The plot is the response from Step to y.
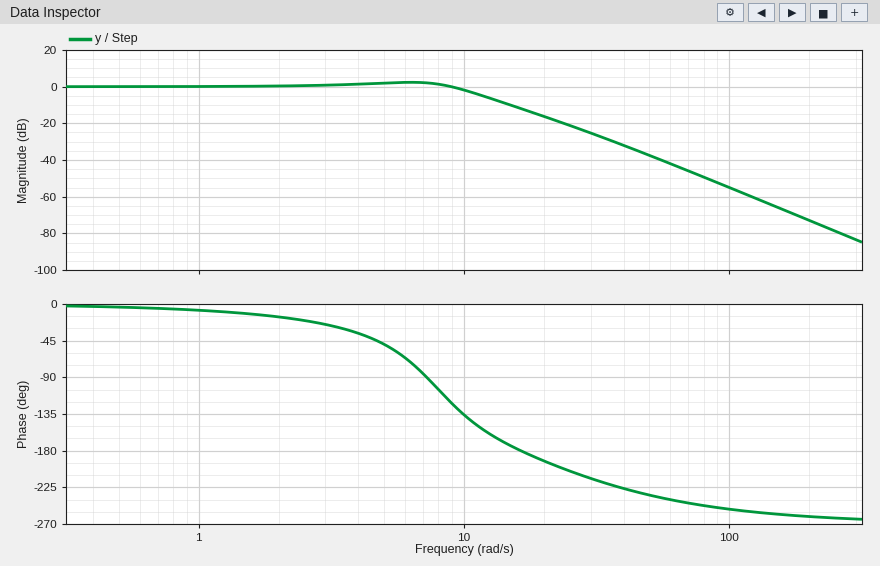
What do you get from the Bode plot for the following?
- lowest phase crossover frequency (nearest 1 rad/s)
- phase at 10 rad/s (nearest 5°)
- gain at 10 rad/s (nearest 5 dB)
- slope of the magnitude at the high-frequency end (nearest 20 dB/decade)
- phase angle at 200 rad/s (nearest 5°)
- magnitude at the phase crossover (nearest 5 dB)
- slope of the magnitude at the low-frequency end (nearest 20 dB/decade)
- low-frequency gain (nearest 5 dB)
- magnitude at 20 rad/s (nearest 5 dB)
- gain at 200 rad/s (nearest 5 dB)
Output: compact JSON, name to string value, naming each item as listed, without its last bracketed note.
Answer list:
{"lowest phase crossover frequency": "16 rad/s", "phase at 10 rad/s": "-135°", "gain at 10 rad/s": "0 dB", "slope of the magnitude at the high-frequency end": "-60 dB/decade", "phase angle at 200 rad/s": "-260°", "magnitude at the phase crossover": "-10 dB", "slope of the magnitude at the low-frequency end": "0 dB/decade", "low-frequency gain": "0 dB", "magnitude at 20 rad/s": "-15 dB", "gain at 200 rad/s": "-75 dB"}
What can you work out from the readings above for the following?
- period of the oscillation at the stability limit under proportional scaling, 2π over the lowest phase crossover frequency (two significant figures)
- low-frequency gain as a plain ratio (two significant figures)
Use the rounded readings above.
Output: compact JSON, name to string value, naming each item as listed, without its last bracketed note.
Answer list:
{"period of the oscillation at the stability limit under proportional scaling, 2π over the lowest phase crossover frequency": "0.39 s", "low-frequency gain as a plain ratio": "1.0"}
